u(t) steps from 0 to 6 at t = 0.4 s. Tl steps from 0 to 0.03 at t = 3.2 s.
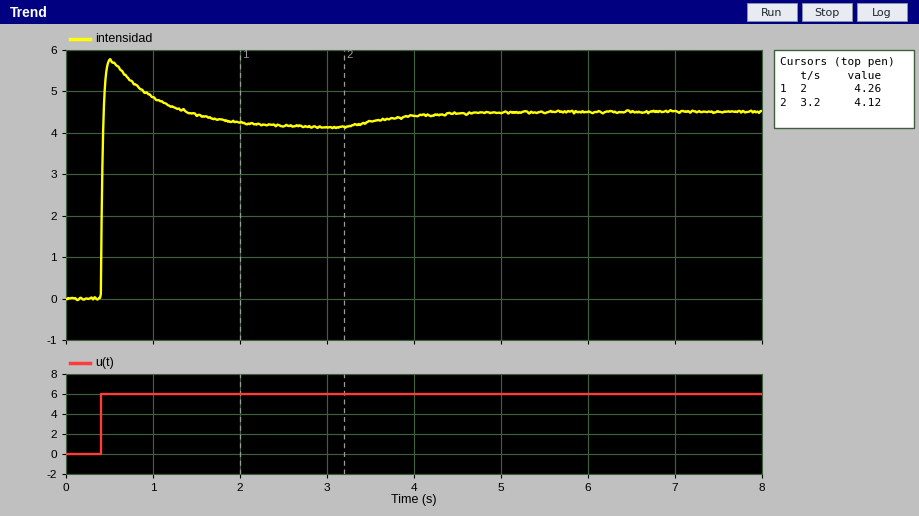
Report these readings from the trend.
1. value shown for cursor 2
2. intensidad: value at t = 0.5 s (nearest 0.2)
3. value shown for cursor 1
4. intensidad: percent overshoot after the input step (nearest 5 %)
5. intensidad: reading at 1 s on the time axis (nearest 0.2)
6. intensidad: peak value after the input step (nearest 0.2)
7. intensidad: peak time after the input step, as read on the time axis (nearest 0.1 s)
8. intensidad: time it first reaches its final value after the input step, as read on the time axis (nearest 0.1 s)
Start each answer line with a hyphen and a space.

- 4.12
- 5.8
- 4.26
- 40 %
- 4.8
- 5.8
- 0.5 s
- 0.4 s
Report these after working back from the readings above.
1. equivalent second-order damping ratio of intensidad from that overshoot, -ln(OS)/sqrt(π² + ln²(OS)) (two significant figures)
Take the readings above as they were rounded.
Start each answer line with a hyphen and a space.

- 0.28
